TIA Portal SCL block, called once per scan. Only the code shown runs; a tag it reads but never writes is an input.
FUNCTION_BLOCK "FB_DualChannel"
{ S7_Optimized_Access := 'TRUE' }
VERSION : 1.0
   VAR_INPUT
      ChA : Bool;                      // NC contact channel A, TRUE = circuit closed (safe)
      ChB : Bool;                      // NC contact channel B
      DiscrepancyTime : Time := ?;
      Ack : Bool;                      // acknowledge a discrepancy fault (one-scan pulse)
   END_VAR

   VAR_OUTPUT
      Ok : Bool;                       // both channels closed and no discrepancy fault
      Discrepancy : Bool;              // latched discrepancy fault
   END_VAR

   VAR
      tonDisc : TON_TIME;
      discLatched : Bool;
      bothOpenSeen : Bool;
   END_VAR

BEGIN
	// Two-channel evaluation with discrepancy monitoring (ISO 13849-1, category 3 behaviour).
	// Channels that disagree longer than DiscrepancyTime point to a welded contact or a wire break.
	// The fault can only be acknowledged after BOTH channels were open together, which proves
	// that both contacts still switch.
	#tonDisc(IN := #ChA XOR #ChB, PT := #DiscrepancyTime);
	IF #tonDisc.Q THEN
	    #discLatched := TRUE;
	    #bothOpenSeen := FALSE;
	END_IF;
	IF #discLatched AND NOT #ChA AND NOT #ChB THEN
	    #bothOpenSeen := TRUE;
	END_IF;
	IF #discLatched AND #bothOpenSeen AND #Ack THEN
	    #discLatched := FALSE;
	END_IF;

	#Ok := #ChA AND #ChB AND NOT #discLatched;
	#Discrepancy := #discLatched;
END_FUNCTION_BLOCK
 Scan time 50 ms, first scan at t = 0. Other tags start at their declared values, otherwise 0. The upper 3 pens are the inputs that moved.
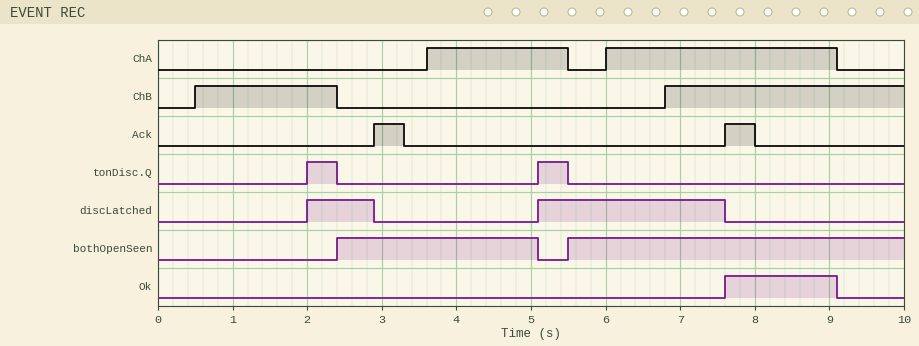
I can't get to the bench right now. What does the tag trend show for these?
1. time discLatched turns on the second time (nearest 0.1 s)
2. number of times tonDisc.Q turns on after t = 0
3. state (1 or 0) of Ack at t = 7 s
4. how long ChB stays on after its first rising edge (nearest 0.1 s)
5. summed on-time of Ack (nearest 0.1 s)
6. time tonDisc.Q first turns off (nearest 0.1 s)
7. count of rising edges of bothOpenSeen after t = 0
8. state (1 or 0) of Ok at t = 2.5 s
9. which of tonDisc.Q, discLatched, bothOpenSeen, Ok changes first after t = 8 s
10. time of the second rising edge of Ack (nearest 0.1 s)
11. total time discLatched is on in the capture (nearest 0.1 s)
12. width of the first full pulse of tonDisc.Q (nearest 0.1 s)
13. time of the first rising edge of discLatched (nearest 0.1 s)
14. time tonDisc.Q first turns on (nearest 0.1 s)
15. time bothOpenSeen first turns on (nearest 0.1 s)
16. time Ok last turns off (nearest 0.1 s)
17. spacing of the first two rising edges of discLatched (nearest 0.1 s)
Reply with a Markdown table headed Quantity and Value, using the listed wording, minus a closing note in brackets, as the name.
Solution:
| Quantity | Value |
|---|---|
| time discLatched turns on the second time | 5.1 s |
| number of times tonDisc.Q turns on after t = 0 | 2 |
| state (1 or 0) of Ack at t = 7 s | 0 |
| how long ChB stays on after its first rising edge | 1.9 s |
| summed on-time of Ack | 0.8 s |
| time tonDisc.Q first turns off | 2.4 s |
| count of rising edges of bothOpenSeen after t = 0 | 2 |
| state (1 or 0) of Ok at t = 2.5 s | 0 |
| which of tonDisc.Q, discLatched, bothOpenSeen, Ok changes first after t = 8 s | Ok |
| time of the second rising edge of Ack | 7.6 s |
| total time discLatched is on in the capture | 3.4 s |
| width of the first full pulse of tonDisc.Q | 0.4 s |
| time of the first rising edge of discLatched | 2.0 s |
| time tonDisc.Q first turns on | 2.0 s |
| time bothOpenSeen first turns on | 2.4 s |
| time Ok last turns off | 9.1 s |
| spacing of the first two rising edges of discLatched | 3.1 s |
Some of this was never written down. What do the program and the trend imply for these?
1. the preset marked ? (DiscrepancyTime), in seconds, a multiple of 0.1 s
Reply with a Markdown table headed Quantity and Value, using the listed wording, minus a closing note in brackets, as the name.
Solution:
| Quantity | Value |
|---|---|
| the preset marked ? (DiscrepancyTime), in seconds, a multiple of 0.1 s | 1.5 s |
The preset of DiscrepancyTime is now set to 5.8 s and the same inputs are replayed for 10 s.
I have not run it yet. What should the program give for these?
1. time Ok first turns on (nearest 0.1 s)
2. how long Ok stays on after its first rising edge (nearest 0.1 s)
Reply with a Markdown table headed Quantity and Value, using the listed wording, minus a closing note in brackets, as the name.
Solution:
| Quantity | Value |
|---|---|
| time Ok first turns on | 6.8 s |
| how long Ok stays on after its first rising edge | 2.3 s |
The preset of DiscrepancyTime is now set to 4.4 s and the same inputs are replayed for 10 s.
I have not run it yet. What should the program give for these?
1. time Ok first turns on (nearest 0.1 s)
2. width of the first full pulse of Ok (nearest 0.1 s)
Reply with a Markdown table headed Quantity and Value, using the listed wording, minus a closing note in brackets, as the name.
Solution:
| Quantity | Value |
|---|---|
| time Ok first turns on | 6.8 s |
| width of the first full pulse of Ok | 2.3 s |
